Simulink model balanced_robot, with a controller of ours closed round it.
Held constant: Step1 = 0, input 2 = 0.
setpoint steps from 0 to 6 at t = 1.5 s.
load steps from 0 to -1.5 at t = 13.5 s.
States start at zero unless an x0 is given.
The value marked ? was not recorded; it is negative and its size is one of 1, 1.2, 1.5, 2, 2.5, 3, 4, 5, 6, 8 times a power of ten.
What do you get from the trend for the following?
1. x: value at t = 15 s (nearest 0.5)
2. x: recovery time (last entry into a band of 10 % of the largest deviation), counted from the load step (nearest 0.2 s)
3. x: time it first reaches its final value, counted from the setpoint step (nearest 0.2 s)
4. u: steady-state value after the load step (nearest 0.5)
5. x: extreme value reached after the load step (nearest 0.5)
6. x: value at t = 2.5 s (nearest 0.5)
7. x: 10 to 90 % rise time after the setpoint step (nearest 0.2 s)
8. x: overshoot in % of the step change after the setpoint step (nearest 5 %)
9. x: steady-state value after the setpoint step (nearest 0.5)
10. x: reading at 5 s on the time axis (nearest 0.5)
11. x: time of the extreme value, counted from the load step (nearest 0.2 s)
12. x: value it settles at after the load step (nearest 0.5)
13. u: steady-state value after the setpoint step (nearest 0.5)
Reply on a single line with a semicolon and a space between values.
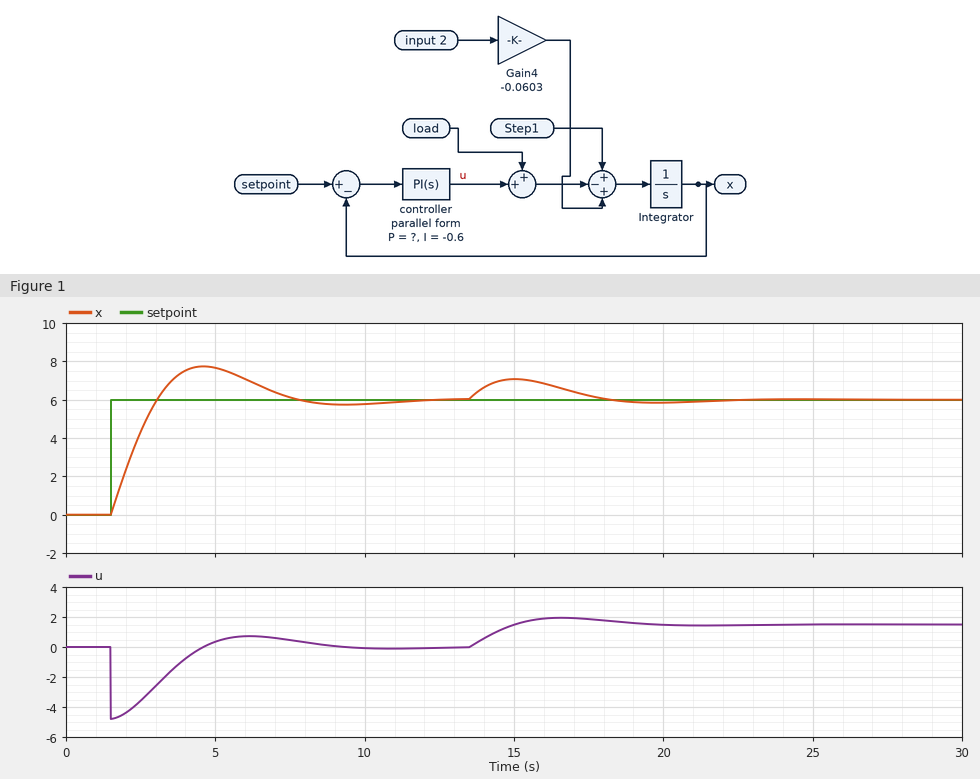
7.0; 7.6 s; 1.6 s; 1.5; 7.0; 4.5; 1.2 s; 30 %; 6.0; 7.5; 1.6 s; 6.0; 0.0
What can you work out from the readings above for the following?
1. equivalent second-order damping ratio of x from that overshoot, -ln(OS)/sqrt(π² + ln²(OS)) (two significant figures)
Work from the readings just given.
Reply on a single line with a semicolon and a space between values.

0.36
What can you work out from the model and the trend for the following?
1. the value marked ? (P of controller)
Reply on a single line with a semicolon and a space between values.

-0.8
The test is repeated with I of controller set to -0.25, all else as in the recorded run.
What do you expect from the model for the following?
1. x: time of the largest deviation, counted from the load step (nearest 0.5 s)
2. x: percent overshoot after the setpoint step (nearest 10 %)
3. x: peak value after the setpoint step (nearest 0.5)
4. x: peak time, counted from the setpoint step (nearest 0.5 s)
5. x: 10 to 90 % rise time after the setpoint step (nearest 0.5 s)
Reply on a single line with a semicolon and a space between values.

2.0 s; 20 %; 7.0; 4.5 s; 1.5 s
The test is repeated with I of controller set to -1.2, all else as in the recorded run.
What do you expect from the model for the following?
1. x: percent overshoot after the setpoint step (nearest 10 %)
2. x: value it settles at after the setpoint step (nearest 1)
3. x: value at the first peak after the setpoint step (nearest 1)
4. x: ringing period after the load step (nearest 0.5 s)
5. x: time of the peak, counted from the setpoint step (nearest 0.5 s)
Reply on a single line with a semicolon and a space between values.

40 %; 6; 8; 6.0 s; 2.5 s
